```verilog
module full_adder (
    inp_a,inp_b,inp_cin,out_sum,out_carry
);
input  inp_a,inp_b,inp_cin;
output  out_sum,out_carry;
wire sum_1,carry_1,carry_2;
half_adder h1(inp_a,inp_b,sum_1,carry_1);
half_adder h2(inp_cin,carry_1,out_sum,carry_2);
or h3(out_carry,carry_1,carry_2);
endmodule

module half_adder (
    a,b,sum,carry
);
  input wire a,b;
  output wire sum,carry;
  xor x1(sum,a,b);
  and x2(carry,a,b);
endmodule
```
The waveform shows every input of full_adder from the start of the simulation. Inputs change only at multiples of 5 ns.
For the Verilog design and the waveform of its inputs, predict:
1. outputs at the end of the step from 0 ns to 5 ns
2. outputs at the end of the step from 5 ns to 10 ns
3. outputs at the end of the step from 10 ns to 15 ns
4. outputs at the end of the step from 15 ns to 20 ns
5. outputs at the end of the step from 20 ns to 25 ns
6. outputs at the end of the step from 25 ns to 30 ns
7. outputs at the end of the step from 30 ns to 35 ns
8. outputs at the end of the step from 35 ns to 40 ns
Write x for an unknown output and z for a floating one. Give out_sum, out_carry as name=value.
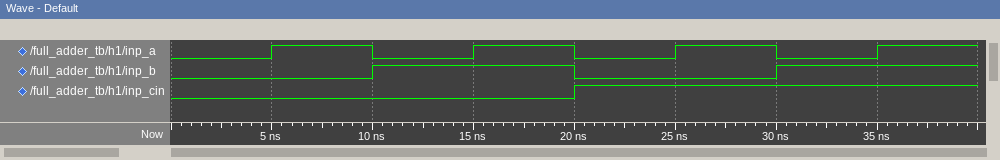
out_sum=0, out_carry=0
out_sum=0, out_carry=0
out_sum=0, out_carry=0
out_sum=1, out_carry=1
out_sum=1, out_carry=0
out_sum=1, out_carry=0
out_sum=1, out_carry=0
out_sum=0, out_carry=1
